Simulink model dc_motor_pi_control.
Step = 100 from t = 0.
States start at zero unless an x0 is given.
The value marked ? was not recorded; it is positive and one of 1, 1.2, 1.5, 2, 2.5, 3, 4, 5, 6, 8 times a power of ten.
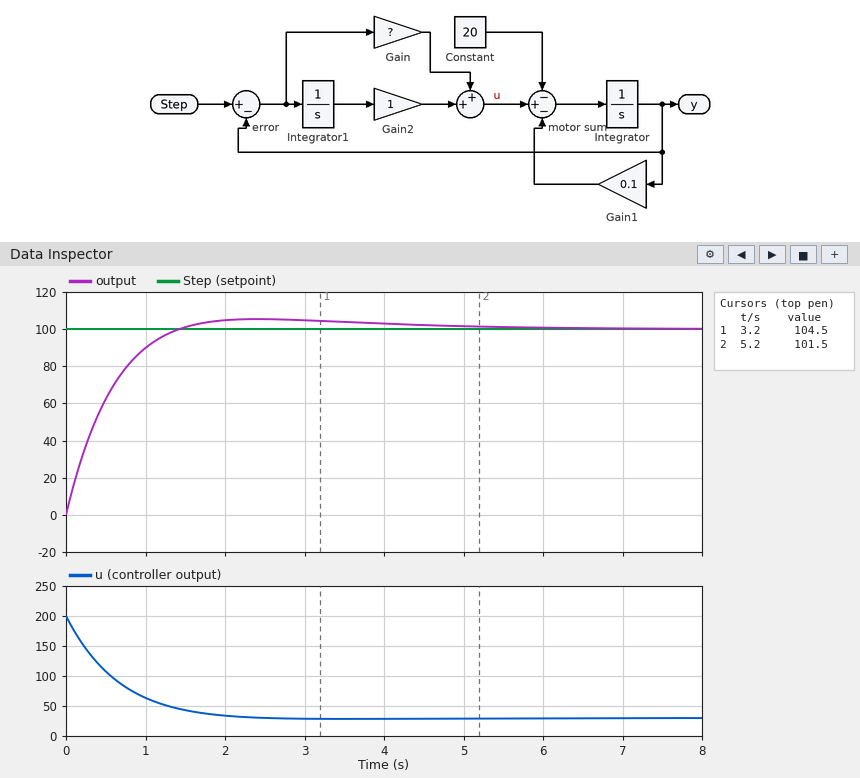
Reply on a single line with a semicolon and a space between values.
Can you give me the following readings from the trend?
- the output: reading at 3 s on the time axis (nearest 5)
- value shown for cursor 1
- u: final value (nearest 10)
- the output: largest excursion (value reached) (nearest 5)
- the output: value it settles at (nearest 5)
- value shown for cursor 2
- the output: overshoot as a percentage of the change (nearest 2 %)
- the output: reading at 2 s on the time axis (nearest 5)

105; 104.5; 30; 105; 100; 101.5; 6 %; 105
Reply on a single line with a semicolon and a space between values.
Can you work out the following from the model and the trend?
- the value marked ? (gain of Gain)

2
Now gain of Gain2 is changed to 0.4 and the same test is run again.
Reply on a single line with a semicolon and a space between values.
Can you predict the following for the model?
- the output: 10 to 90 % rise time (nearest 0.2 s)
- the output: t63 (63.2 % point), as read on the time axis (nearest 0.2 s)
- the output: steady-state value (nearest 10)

1.4 s; 0.6 s; 100
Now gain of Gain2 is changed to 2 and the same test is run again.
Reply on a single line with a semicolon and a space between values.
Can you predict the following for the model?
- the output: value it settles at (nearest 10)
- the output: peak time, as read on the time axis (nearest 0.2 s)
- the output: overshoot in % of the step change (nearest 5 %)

100; 1.8 s; 15 %
